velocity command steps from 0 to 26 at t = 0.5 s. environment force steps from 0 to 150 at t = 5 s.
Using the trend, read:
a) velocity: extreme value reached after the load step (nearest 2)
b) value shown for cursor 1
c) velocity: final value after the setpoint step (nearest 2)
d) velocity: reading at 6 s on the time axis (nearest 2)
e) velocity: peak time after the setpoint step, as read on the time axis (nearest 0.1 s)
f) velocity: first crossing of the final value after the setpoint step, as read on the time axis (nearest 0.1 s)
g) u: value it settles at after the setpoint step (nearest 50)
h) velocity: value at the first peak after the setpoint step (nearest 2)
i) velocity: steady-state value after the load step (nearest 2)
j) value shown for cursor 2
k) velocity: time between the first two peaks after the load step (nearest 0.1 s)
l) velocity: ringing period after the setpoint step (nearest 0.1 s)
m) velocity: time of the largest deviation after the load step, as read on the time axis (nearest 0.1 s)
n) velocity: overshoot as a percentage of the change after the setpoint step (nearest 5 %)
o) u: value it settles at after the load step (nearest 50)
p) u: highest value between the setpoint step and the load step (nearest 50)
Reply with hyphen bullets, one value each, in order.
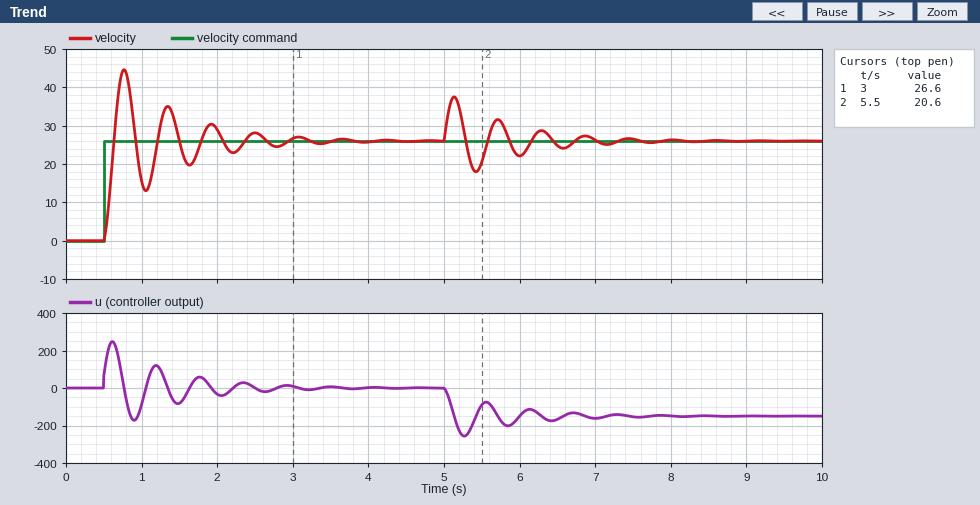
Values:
- 38
- 26.6
- 26
- 22
- 0.8 s
- 0.6 s
- 0
- 44
- 26
- 20.6
- 0.6 s
- 0.6 s
- 5.1 s
- 70 %
- -150
- 250
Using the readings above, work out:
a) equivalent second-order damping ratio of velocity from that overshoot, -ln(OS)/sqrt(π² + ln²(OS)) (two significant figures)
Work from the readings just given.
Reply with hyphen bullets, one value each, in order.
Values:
- 0.11
